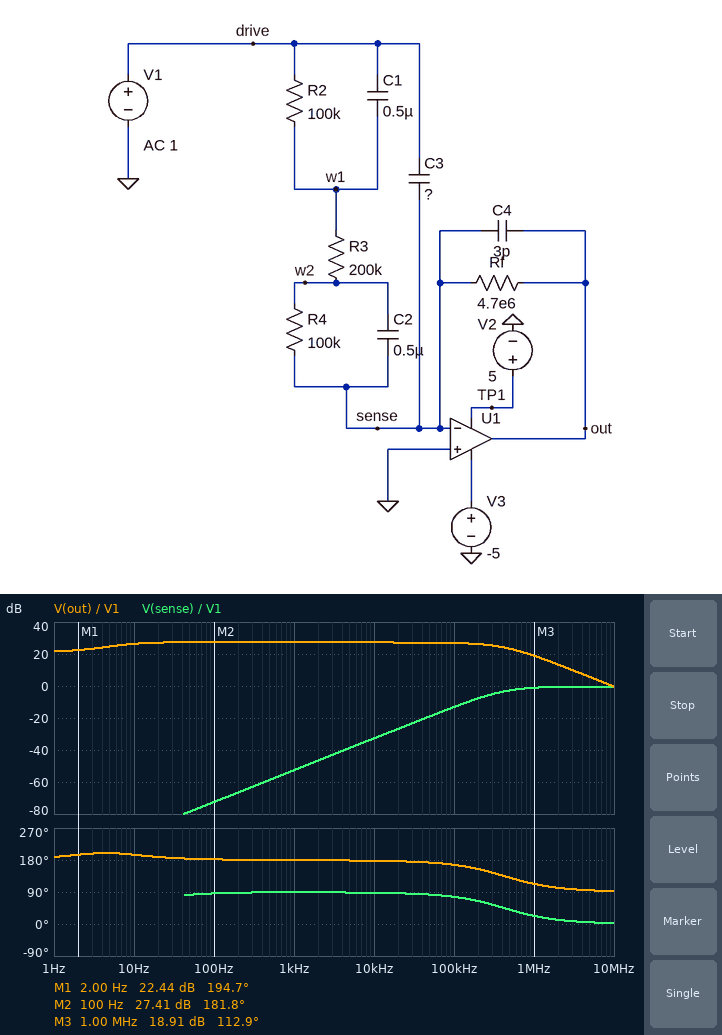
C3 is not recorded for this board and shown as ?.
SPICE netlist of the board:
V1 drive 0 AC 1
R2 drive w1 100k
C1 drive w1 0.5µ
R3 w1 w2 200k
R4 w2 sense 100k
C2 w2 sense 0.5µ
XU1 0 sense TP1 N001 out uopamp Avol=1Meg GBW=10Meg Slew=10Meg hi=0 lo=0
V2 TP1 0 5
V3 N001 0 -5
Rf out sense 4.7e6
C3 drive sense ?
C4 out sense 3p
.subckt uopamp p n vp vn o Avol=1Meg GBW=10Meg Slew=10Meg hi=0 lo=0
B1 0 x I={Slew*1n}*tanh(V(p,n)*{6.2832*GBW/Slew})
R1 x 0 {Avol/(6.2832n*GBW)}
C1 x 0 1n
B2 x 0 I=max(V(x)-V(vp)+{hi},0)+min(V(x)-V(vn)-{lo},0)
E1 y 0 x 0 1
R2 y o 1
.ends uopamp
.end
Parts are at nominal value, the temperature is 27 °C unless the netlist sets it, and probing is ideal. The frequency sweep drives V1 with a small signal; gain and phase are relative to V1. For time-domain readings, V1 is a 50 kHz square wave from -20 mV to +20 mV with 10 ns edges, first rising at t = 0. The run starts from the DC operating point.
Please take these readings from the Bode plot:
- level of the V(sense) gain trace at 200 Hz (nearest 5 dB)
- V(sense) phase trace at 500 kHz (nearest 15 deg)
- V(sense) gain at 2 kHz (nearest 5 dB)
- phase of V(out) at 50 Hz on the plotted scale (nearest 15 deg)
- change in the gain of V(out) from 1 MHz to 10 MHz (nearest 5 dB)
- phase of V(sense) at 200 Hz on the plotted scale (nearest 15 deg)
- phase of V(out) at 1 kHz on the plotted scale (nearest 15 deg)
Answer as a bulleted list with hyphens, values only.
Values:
- -65 dB
- 45 deg
- -45 dB
- 180 deg
- -20 dB
- 90 deg
- 180 deg
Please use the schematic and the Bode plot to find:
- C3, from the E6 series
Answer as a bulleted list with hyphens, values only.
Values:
- 68 pF
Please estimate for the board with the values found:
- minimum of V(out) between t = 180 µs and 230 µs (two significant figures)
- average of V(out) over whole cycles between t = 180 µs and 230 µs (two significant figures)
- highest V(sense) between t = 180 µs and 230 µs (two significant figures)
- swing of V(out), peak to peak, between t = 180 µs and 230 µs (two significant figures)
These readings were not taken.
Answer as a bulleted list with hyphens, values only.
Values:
- -690 mV
- -230 mV
- 38 mV
- 920 mV
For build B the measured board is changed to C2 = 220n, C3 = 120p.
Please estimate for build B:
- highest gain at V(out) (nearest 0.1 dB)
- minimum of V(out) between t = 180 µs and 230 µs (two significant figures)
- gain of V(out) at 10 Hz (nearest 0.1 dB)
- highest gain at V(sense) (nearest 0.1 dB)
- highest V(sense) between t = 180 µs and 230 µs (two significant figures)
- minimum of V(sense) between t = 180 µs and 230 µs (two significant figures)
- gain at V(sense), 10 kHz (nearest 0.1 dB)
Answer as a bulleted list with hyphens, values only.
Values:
- 31.9 dB
- -1.1 V
- 25.3 dB
- -0.2 dB
- 39 mV
- -39 mV
- -29.9 dB
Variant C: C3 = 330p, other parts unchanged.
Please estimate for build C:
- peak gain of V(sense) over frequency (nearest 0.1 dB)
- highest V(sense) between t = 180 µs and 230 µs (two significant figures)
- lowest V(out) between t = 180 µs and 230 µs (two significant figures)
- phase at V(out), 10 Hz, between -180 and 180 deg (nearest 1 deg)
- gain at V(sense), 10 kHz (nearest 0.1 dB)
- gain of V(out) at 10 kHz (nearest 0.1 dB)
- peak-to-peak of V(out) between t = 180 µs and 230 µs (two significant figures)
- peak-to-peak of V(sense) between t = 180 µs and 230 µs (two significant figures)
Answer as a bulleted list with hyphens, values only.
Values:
- -0.1 dB
- 41 mV
- -2.5 V
- -165 deg
- -22.1 dB
- 37.9 dB
- 4.5 V
- 82 mV
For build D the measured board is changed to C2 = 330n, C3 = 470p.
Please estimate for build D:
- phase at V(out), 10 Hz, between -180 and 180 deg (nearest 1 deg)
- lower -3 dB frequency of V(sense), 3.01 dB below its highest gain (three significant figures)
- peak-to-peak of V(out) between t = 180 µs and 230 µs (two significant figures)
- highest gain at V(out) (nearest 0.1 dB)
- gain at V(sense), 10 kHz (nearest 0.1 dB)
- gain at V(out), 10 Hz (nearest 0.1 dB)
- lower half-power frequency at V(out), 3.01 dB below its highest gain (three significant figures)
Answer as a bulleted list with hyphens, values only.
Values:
- -163 deg
- 54.6 kHz
- 6.0 V
- 43.7 dB
- -19.0 dB
- 25.9 dB
- 9.37 kHz
